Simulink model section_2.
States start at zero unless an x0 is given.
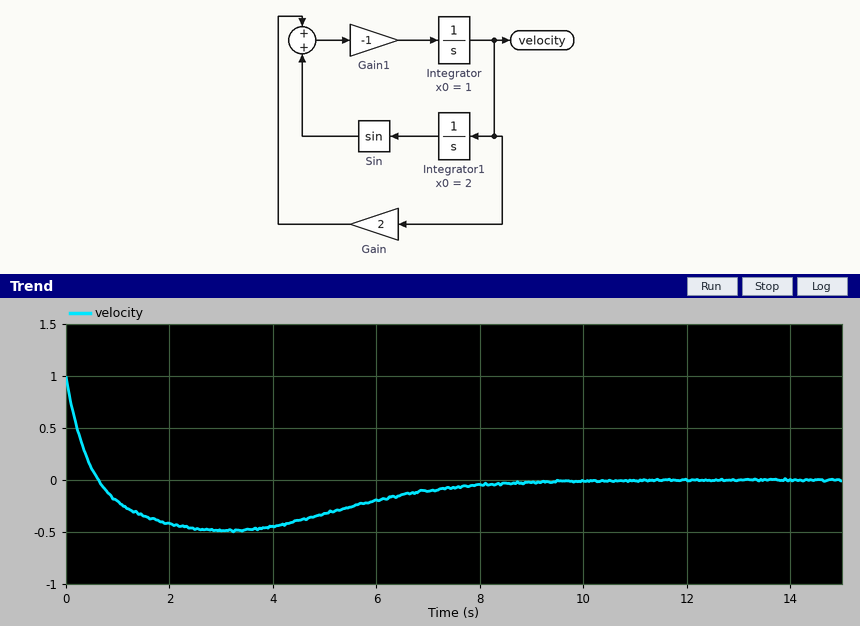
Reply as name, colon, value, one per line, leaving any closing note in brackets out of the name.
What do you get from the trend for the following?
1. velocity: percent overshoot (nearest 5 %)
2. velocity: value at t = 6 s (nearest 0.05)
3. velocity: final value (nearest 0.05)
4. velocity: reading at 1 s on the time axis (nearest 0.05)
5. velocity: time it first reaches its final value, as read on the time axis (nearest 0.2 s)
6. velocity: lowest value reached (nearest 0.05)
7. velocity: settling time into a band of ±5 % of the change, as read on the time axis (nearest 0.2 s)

velocity: percent overshoot: 50 %
velocity: value at t = 6 s: -0.20
velocity: final value: 0.00
velocity: reading at 1 s on the time axis: -0.20
velocity: time it first reaches its final value, as read on the time axis: 0.6 s
velocity: lowest value reached: -0.50
velocity: settling time into a band of ±5 % of the change, as read on the time axis: 8.0 s
